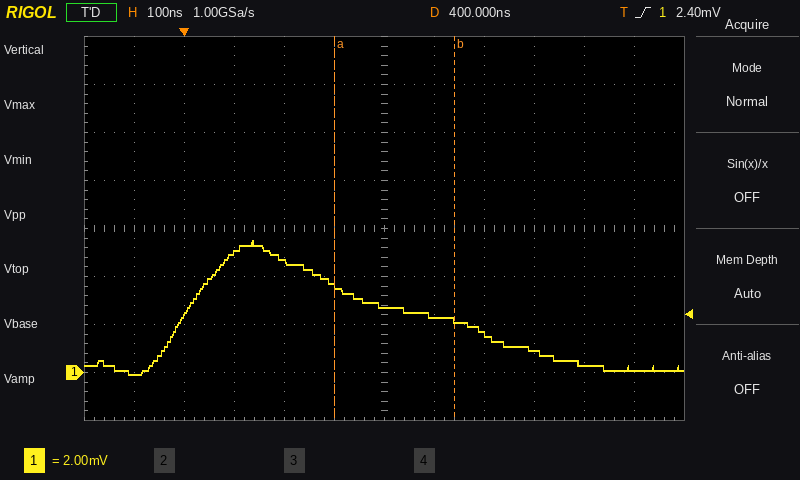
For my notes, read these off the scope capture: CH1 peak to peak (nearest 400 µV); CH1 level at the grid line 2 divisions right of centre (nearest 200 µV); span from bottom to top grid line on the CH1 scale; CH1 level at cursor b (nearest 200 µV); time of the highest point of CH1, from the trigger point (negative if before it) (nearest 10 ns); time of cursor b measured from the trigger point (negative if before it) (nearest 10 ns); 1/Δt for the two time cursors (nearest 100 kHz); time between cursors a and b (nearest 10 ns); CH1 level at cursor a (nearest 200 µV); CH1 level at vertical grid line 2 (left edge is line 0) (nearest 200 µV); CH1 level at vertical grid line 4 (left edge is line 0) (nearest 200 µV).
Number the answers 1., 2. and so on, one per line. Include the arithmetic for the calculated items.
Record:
1. 5.6 mV
2. 1.6 mV
3. 16 mV
4. 2.2 mV
5. +140 ns
6. +540 ns
7. 1 / 240 ns ≈ 4.2 MHz
8. 240 ns
9. 3.6 mV
10. 2.4 mV
11. 4.6 mV
